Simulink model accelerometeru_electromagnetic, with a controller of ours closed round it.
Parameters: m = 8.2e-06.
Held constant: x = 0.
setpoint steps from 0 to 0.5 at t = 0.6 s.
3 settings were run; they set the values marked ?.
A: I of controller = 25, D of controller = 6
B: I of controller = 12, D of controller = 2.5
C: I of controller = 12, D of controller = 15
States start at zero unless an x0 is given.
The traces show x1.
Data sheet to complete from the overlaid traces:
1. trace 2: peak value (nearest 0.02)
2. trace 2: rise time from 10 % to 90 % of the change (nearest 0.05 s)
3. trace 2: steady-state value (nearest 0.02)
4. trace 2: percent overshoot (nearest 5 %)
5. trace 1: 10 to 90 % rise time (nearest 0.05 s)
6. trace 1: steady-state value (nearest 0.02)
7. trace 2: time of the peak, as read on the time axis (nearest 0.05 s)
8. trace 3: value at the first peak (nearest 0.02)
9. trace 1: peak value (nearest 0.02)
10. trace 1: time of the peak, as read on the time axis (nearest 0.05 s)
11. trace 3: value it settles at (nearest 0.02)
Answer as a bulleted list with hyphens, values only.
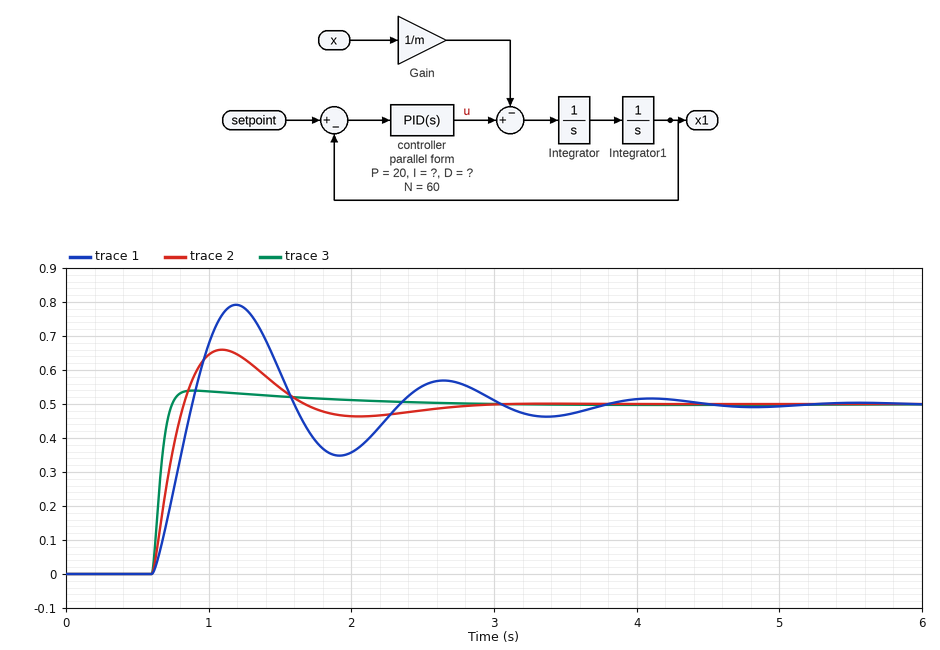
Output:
- 0.66
- 0.15 s
- 0.50
- 30 %
- 0.20 s
- 0.50
- 1.10 s
- 0.54
- 0.80
- 1.20 s
- 0.50
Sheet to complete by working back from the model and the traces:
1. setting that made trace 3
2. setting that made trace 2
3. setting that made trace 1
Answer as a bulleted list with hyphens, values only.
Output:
- C
- A
- B
